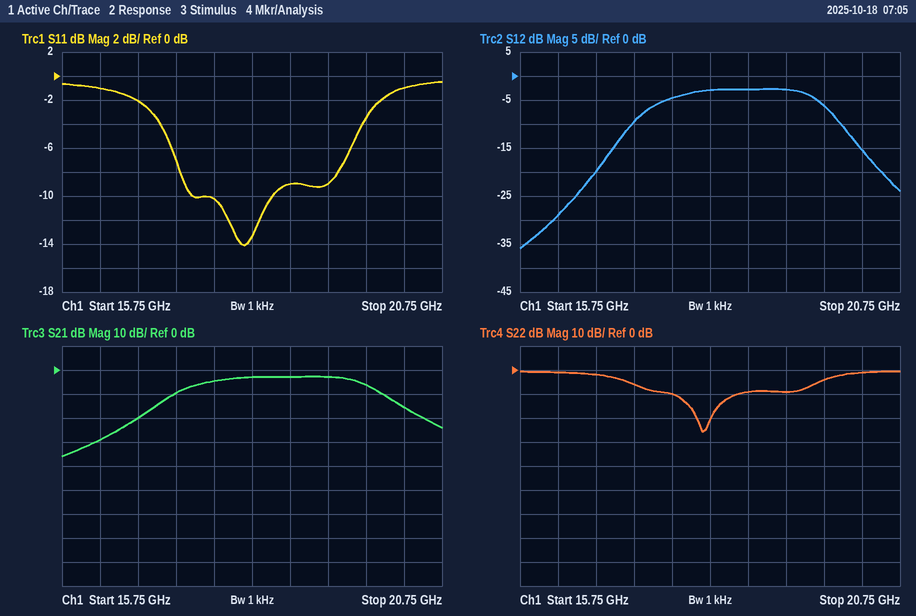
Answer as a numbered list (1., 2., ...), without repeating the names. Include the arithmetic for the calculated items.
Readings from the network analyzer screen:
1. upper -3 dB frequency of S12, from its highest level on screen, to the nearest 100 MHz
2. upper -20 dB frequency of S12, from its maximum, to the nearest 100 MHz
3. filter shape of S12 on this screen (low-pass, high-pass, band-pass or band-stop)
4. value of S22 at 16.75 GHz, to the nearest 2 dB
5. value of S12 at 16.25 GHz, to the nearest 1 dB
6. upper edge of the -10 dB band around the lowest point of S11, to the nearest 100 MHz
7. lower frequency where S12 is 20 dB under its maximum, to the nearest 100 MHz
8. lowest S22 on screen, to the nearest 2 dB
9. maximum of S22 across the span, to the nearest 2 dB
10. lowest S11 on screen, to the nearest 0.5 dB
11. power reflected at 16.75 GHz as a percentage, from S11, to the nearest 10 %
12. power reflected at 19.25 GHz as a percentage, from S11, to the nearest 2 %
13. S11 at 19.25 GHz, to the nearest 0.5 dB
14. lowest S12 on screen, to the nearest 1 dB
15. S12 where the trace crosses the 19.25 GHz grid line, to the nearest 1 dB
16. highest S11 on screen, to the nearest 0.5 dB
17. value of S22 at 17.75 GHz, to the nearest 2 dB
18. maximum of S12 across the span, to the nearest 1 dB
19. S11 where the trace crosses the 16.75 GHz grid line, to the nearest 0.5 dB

1. 19.7 GHz
2. 20.7 GHz
3. band-pass
4. -2 dB
5. -29 dB
6. 18.5 GHz
7. 16.6 GHz
8. -26 dB
9. 0 dB
10. -14.0 dB
11. 10^(-2/10) ≈ 63.1 %, so 60 % to the nearest 10 %
12. 10^(-9/10) ≈ 12.6 %, so 12 % to the nearest 2 %
13. -9.0 dB
14. -36 dB
15. -3 dB
16. -0.5 dB
17. -10 dB
18. -3 dB
19. -2.0 dB
